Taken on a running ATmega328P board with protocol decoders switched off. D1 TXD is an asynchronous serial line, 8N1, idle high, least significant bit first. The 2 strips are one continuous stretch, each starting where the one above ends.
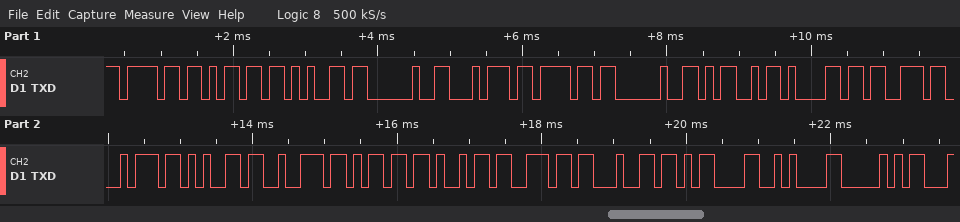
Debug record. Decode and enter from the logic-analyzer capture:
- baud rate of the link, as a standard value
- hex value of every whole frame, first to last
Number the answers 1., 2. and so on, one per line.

1. 9600 baud
2. 6F 6D 65 20 74 6F 20 4D 61 73 74 65 72 6D 69 6E 64 0D 0A 50
